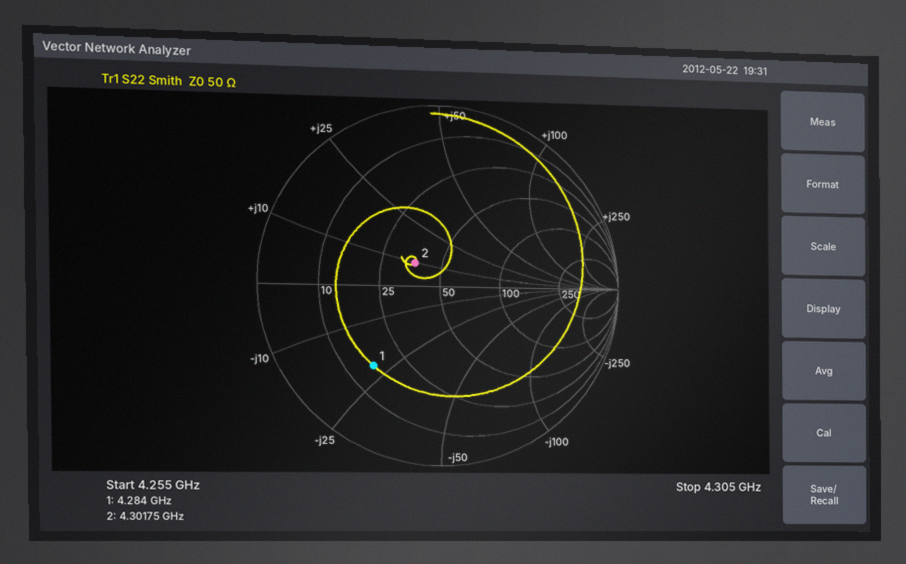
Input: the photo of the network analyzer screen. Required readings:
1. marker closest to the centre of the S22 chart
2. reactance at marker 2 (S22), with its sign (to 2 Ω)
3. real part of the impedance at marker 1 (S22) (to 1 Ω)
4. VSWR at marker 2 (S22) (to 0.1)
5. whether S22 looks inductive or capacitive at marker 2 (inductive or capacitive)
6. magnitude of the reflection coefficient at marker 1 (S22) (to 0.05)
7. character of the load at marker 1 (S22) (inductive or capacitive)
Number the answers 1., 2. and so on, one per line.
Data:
1. marker 2
2. +10 Ω
3. 16 Ω
4. 1.5
5. inductive
6. 0.60
7. capacitive
